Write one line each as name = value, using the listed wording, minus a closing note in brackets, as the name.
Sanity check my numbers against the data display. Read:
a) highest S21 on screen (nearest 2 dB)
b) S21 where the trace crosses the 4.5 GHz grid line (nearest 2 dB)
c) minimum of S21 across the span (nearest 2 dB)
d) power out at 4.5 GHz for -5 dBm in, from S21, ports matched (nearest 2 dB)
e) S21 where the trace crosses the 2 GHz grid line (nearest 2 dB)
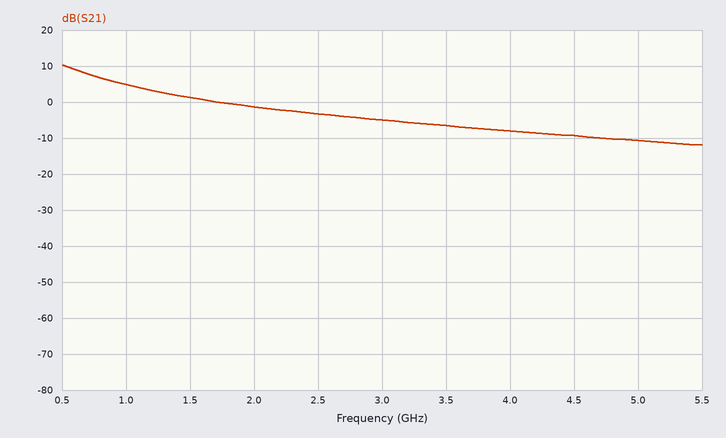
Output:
highest S21 on screen = 10 dB
S21 where the trace crosses the 4.5 GHz grid line = -10 dB
minimum of S21 across the span = -12 dB
power out at 4.5 GHz for -5 dBm in, from S21, ports matched = -14 dBm
S21 where the trace crosses the 2 GHz grid line = -2 dB
